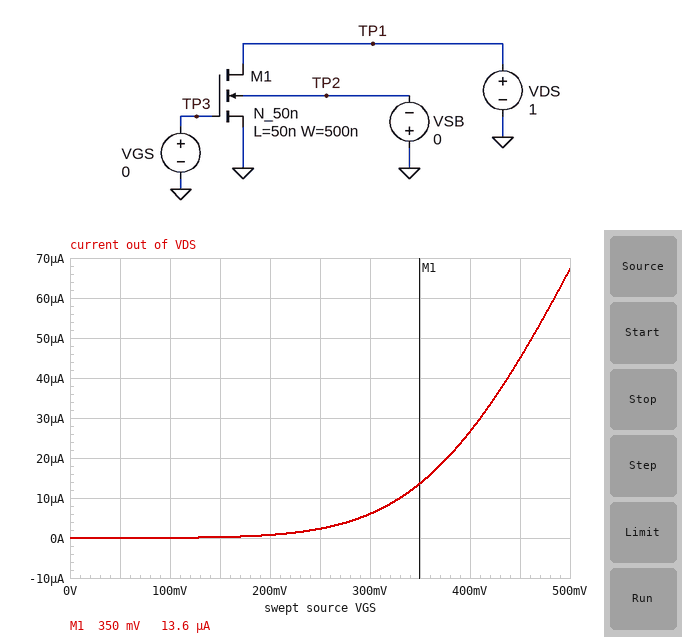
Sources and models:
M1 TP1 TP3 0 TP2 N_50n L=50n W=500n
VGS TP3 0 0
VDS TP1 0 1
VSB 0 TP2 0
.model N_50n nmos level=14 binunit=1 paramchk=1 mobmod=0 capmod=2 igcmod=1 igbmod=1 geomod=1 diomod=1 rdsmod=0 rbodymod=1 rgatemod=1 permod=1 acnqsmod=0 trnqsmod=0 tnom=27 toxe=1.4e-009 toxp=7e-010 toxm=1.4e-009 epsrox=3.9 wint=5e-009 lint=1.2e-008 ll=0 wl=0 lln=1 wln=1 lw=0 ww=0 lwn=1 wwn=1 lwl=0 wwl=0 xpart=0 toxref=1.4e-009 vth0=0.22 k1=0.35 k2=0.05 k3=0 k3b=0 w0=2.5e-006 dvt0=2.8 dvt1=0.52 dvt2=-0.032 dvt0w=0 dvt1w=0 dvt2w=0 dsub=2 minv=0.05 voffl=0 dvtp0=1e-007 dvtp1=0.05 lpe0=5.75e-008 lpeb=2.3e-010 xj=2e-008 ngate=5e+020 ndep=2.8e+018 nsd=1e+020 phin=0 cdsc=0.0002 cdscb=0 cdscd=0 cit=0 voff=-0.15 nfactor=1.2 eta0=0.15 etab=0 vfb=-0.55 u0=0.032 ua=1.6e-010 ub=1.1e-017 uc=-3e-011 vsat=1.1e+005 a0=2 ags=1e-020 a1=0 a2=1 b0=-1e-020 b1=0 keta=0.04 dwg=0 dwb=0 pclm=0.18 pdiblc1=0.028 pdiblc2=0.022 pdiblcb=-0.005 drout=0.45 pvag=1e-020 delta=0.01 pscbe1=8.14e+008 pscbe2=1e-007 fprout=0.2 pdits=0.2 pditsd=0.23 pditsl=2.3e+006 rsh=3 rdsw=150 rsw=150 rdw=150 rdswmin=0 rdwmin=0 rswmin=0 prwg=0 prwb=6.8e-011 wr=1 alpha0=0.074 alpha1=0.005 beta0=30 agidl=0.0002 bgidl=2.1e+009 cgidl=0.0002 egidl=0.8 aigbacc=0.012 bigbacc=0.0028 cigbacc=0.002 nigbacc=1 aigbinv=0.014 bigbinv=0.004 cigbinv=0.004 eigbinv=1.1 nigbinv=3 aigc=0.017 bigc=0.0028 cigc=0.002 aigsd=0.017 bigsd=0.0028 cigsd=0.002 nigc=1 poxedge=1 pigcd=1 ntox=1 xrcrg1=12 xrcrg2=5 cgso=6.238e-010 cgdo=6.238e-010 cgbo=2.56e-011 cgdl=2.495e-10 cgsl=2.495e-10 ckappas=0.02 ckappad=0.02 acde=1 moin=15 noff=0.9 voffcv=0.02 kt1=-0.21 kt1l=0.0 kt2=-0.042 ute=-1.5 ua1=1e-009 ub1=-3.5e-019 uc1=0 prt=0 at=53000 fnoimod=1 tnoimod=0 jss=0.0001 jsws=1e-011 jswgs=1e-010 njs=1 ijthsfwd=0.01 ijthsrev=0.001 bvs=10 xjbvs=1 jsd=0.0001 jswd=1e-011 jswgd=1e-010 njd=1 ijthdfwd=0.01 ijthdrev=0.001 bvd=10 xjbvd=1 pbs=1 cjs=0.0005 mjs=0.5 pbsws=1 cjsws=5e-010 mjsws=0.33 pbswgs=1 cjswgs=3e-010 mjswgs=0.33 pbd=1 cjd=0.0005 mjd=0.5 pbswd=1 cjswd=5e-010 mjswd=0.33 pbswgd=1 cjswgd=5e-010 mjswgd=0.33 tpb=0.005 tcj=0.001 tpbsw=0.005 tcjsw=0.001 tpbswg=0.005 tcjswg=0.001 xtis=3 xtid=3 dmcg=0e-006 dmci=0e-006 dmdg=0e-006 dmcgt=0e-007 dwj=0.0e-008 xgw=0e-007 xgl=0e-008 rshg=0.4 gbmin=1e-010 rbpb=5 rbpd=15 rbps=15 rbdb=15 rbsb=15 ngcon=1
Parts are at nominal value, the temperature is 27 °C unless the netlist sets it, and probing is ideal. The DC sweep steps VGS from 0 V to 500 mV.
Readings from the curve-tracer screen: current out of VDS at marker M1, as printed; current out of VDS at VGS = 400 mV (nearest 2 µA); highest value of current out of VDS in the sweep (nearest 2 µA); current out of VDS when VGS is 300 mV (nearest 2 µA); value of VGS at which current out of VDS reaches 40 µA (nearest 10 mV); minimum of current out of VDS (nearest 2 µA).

13.6 µA
26 µA
68 µA
6 µA
440 mV
0 A
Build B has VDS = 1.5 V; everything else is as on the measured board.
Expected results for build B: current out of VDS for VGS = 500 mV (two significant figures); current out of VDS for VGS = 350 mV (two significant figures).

82 µA
18 µA
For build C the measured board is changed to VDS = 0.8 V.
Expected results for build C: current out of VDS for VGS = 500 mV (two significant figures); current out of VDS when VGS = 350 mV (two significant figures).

62 µA
12 µA
